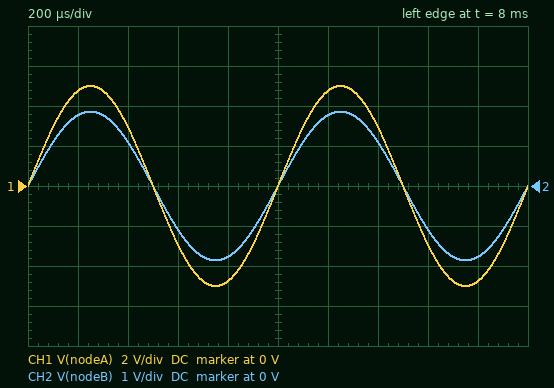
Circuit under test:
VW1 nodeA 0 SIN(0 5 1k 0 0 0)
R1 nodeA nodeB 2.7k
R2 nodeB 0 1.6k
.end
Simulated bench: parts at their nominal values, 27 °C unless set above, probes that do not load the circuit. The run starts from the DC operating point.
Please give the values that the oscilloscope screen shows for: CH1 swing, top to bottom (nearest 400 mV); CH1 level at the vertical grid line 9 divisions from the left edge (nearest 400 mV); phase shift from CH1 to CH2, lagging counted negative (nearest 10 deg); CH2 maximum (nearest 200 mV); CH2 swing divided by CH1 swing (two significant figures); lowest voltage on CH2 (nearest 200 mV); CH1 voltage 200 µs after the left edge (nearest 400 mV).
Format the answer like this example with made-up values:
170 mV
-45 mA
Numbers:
10.0 V
-4.8 V
0 deg
1.8 V
0.37
-1.8 V
4.8 V
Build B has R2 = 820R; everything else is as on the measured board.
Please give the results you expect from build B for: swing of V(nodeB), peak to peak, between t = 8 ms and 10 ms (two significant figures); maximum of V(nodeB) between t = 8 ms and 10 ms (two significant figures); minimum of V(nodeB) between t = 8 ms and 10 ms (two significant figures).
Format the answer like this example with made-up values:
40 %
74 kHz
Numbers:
2.3 V
1.2 V
-1.2 V
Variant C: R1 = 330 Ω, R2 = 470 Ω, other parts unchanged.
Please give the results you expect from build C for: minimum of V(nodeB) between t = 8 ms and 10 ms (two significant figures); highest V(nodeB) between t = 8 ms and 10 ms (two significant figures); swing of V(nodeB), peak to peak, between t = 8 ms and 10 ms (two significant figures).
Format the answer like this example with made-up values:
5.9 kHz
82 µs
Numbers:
-2.9 V
2.9 V
5.9 V
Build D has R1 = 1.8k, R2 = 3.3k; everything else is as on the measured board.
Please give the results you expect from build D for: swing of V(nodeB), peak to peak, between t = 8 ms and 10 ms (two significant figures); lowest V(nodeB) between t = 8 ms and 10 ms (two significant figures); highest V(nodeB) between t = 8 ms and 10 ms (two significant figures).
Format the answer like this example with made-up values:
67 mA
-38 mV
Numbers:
6.5 V
-3.2 V
3.2 V
